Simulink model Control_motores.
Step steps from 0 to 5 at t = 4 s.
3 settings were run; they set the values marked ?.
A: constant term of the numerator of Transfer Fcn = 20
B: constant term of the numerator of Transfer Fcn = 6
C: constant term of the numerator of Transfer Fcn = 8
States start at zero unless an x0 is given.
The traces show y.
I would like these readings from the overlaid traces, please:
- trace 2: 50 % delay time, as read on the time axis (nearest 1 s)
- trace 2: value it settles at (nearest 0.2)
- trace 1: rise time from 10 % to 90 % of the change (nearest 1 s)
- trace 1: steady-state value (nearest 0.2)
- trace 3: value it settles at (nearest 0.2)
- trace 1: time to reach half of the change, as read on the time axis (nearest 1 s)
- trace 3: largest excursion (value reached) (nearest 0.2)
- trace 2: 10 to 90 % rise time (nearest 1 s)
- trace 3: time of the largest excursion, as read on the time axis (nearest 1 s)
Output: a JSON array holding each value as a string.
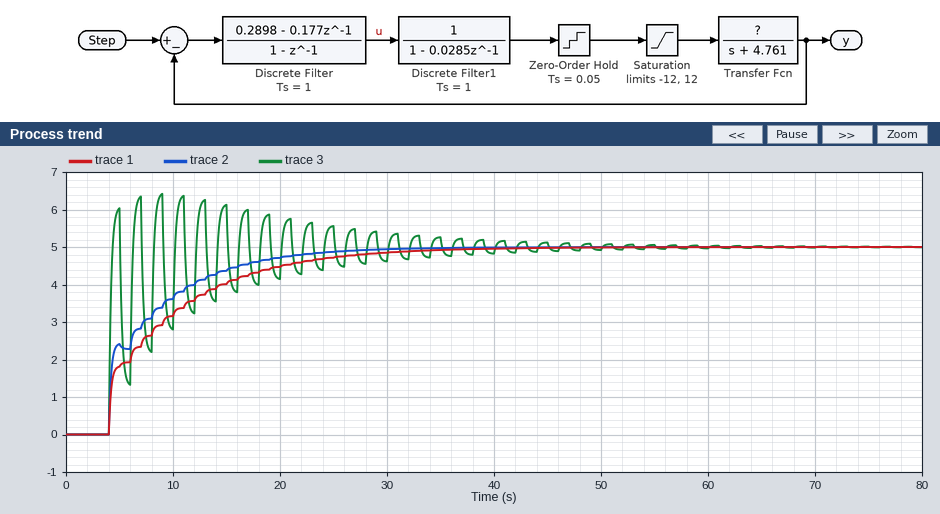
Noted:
["6 s", "5.0", "16 s", "5.0", "5.0", "7 s", "6.4", "12 s", "9 s"]
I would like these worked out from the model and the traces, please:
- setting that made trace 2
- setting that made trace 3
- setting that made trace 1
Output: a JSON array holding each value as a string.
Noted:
["C", "A", "B"]
